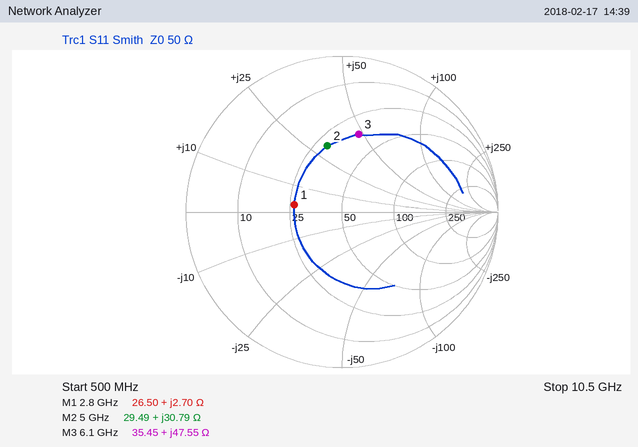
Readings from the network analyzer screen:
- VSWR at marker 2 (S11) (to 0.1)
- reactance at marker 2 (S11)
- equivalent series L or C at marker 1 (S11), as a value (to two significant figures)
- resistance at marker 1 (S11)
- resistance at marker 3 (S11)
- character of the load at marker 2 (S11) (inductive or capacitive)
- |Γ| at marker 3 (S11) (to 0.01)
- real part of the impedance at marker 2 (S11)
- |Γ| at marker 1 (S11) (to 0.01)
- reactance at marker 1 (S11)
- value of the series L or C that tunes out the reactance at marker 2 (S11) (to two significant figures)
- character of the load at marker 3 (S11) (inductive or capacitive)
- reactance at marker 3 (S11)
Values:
2.5
+30.79 Ω
150 pH
26.50 Ω
35.45 Ω
inductive
0.51
29.49 Ω
0.31
+2.70 Ω
1.0 pF
inductive
+47.55 Ω
